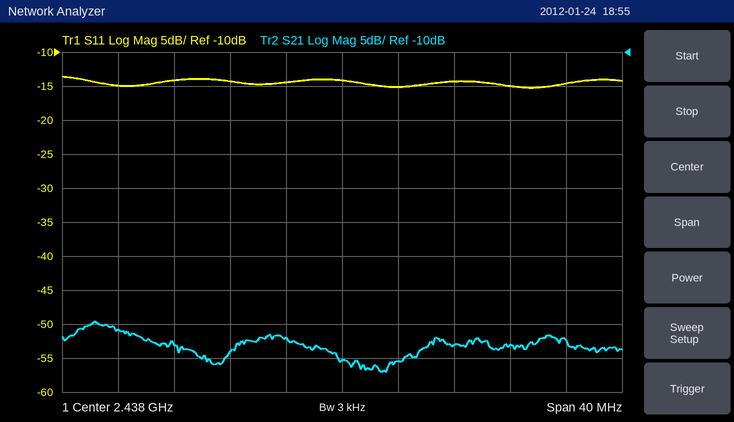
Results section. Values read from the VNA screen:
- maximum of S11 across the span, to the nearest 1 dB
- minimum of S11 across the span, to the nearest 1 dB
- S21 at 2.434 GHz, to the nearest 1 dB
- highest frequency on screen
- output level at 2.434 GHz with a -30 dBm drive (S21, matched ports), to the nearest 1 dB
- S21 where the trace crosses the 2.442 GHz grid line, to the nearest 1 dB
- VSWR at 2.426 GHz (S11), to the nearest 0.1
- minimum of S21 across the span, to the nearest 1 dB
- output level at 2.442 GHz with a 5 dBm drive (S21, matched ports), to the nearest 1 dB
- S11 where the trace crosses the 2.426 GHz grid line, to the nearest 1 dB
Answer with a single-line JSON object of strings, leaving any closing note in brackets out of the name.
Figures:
{"maximum of S11 across the span, to the nearest 1 dB": "-14 dB", "minimum of S11 across the span, to the nearest 1 dB": "-15 dB", "S21 at 2.434 GHz, to the nearest 1 dB": "-52 dB", "highest frequency on screen": "2.458 GHz", "output level at 2.434 GHz with a -30 dBm drive (S21, matched ports), to the nearest 1 dB": "-82 dBm", "S21 where the trace crosses the 2.442 GHz grid line, to the nearest 1 dB": "-55 dB", "VSWR at 2.426 GHz (S11), to the nearest 0.1": "1.5", "minimum of S21 across the span, to the nearest 1 dB": "-57 dB", "output level at 2.442 GHz with a 5 dBm drive (S21, matched ports), to the nearest 1 dB": "-50 dBm", "S11 where the trace crosses the 2.426 GHz grid line, to the nearest 1 dB": "-14 dB"}
